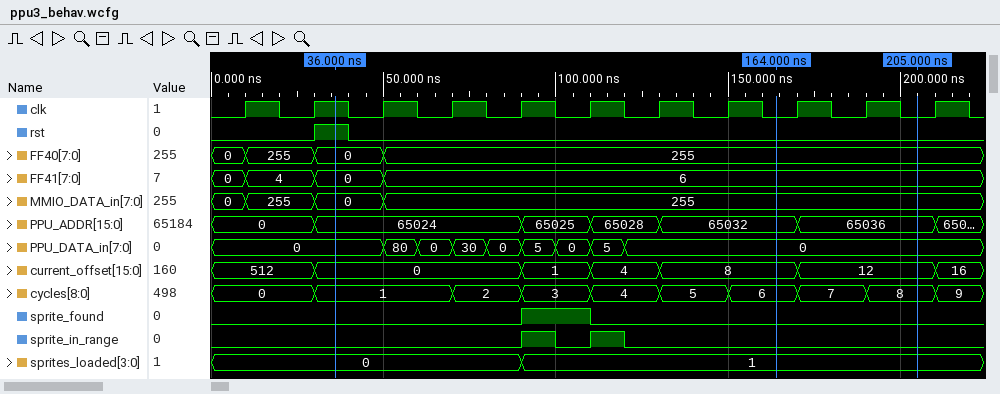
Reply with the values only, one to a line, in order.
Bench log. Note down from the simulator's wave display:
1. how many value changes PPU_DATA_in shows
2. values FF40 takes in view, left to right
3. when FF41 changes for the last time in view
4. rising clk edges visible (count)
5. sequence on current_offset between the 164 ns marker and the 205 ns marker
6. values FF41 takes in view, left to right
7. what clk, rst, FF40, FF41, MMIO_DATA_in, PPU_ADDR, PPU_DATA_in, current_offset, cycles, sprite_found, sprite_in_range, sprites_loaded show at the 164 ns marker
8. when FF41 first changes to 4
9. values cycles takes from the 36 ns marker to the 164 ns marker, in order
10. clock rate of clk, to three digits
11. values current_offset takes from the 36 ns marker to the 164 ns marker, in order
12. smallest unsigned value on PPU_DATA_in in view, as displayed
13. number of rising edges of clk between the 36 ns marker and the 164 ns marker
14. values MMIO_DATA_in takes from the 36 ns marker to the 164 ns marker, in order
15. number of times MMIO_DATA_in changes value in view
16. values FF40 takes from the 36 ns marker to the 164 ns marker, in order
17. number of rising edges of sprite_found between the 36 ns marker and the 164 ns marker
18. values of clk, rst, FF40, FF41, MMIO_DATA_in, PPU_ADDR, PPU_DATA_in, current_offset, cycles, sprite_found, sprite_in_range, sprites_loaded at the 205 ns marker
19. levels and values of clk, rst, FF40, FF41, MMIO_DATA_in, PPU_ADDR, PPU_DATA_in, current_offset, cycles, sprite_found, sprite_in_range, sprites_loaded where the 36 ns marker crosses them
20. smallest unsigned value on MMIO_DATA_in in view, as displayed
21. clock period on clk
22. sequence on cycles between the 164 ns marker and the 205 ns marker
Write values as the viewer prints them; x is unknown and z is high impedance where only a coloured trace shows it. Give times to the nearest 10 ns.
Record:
8
0, 255, 0, 255
50 ns
11
8, 12
0, 4, 0, 6
clk=0, rst=0, FF40=255, FF41=6, MMIO_DATA_in=255, PPU_ADDR=65032, PPU_DATA_in=0, current_offset=8, cycles=6, sprite_found=0, sprite_in_range=0, sprites_loaded=1
10 ns
1, 2, 3, 4, 5, 6
50.0 MHz
0, 1, 4, 8
0
6
0, 255
3
0, 255
1
clk=0, rst=0, FF40=255, FF41=6, MMIO_DATA_in=255, PPU_ADDR=65036, PPU_DATA_in=0, current_offset=12, cycles=8, sprite_found=0, sprite_in_range=0, sprites_loaded=1
clk=1, rst=1, FF40=0, FF41=0, MMIO_DATA_in=0, PPU_ADDR=65024, PPU_DATA_in=0, current_offset=0, cycles=1, sprite_found=0, sprite_in_range=0, sprites_loaded=0
0
20 ns
6, 7, 8
